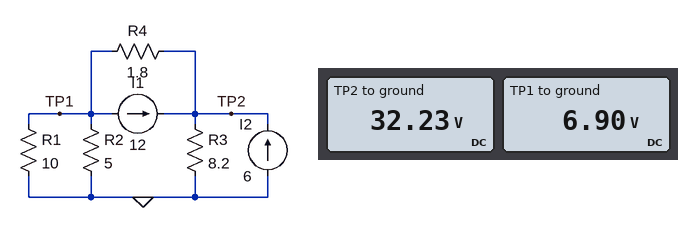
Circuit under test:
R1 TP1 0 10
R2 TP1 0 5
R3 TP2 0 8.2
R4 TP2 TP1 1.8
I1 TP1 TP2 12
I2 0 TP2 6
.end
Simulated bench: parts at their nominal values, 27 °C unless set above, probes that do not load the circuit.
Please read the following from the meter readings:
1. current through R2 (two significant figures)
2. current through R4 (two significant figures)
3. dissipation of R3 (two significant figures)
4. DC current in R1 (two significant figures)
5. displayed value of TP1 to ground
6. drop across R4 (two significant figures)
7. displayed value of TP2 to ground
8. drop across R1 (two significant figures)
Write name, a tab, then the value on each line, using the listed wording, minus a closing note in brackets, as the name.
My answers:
current through R2	1.4 A
current through R4	14 A
dissipation of R3	130 W
DC current in R1	690 mA
displayed value of TP1 to ground	6.90 V
drop across R4	25 V
displayed value of TP2 to ground	32.23 V
drop across R1	6.9 V
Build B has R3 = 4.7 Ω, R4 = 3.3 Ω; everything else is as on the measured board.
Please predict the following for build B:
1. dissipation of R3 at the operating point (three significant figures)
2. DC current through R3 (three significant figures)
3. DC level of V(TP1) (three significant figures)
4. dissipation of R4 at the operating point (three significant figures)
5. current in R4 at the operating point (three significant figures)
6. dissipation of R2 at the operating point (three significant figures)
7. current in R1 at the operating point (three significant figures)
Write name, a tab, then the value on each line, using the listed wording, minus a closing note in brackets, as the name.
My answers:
dissipation of R3 at the operating point	231 W
DC current through R3	7.01 A
DC level of V(TP1)	-3.35 V
dissipation of R4 at the operating point	399 W
current in R4 at the operating point	11.0 A
dissipation of R2 at the operating point	2.25 W
current in R1 at the operating point	335 mA
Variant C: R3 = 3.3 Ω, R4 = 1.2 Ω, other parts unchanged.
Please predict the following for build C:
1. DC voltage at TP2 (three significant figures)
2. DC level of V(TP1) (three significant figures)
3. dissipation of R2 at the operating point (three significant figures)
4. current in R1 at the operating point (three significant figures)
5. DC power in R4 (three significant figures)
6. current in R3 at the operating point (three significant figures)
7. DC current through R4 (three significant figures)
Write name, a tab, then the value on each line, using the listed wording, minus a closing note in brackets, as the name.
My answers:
DC voltage at TP2	17.5 V
DC level of V(TP1)	2.30 V
dissipation of R2 at the operating point	1.06 W
current in R1 at the operating point	230 mA
DC power in R4	193 W
current in R3 at the operating point	5.31 A
DC current through R4	12.7 A
